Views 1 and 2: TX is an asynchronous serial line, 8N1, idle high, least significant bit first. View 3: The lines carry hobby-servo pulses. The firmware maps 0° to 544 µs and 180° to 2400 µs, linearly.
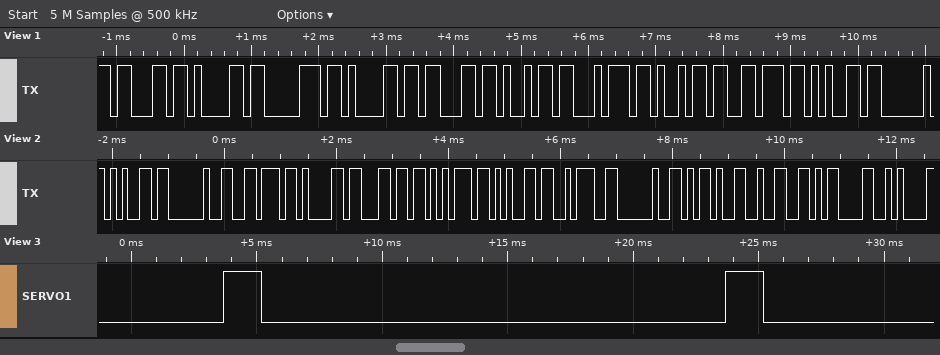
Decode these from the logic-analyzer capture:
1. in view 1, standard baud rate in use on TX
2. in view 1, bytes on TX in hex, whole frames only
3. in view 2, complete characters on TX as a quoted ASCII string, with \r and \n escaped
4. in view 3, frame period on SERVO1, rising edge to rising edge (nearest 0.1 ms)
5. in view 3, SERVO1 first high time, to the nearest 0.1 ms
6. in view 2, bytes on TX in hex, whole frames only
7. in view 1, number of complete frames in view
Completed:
9600 baud
0x63 0x61 0x70 0x61 0x63 0x69 0x74 0x69 0x76 0x65
"e value: -2\r\n"
20.0 ms
1.5 ms
65 20 76 61 6C 75 65 3A 20 2D 32 0D 0A
10
